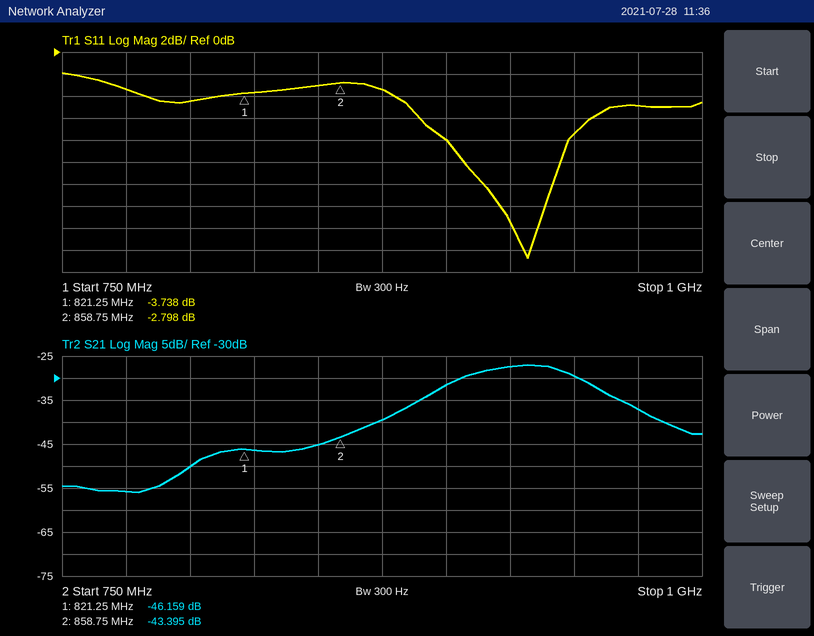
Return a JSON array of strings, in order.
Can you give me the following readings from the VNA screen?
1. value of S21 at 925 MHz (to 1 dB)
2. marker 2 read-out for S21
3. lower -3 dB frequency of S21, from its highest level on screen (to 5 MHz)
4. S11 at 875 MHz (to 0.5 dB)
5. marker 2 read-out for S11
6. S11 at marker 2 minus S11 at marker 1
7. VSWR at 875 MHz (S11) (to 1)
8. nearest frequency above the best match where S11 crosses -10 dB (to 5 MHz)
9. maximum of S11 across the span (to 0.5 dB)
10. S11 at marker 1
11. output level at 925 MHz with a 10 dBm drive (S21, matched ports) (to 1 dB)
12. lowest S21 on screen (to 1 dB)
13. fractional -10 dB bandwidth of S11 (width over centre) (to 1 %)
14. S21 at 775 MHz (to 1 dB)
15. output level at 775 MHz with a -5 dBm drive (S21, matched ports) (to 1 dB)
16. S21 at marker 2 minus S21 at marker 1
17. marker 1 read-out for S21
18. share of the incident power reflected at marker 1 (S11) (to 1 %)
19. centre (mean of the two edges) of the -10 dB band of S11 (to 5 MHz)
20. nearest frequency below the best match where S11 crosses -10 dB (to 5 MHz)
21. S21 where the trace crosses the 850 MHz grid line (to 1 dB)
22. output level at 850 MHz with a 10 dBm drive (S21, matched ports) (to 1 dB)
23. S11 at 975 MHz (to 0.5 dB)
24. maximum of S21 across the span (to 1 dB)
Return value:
["-27 dB", "-43.395 dB", "905 MHz", "-3.5 dB", "-2.798 dB", "0.940 dB", "5", "945 MHz", "-2.0 dB", "-3.738 dB", "-17 dBm", "-56 dB", "4 %", "-56 dB", "-61 dBm", "2.764 dB", "-46.159 dB", "42 %", "925 MHz", "905 MHz", "-45 dB", "-35 dBm", "-5.0 dB", "-27 dB"]
